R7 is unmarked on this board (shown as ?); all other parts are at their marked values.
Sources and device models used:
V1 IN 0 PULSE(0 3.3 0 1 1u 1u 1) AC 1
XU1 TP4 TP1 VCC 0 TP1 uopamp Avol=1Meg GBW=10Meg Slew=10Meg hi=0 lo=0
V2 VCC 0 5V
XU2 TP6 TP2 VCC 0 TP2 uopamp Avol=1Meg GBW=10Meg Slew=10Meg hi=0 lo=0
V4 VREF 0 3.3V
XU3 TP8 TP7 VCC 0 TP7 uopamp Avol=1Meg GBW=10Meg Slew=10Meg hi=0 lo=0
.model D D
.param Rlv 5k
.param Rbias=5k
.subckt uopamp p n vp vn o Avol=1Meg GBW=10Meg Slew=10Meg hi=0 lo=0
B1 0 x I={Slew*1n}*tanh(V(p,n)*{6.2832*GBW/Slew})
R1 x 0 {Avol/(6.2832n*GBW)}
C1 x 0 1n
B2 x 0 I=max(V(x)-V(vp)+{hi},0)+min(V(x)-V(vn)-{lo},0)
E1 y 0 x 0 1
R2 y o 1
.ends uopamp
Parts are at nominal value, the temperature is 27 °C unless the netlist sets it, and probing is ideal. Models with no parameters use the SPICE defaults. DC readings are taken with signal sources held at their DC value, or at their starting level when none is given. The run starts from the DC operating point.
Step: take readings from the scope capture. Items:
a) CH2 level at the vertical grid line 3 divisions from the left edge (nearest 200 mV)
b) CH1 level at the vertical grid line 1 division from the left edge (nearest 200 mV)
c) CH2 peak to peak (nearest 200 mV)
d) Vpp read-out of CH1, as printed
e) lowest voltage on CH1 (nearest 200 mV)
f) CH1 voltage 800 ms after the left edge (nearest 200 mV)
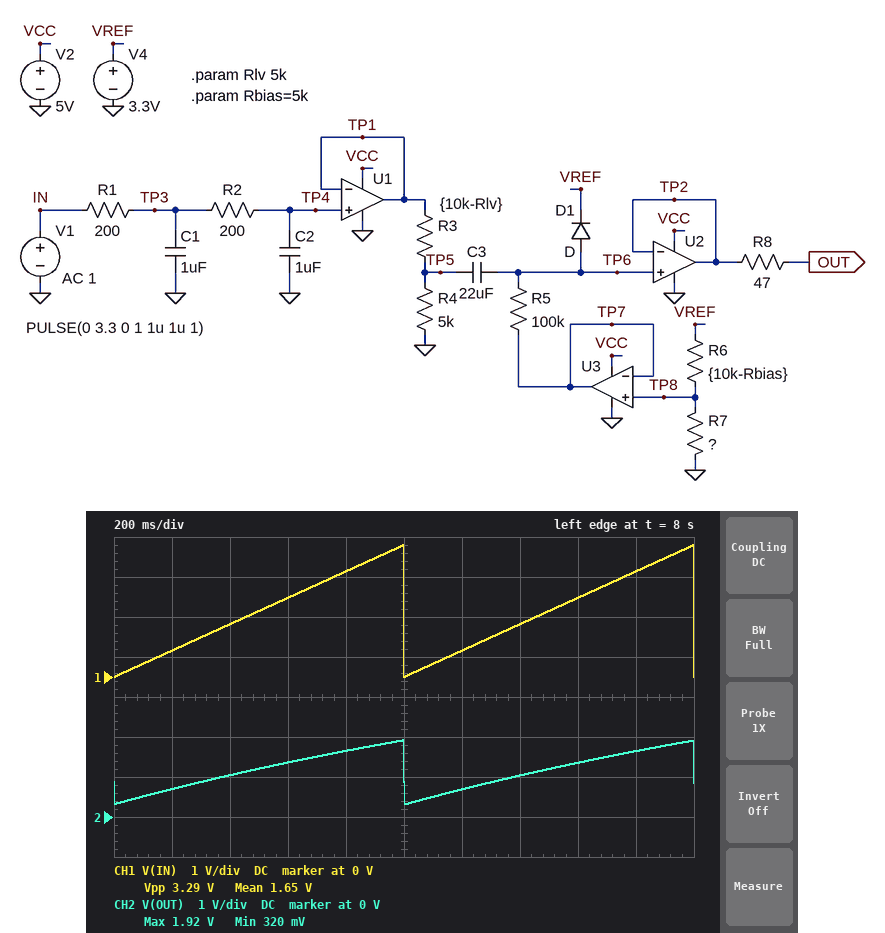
1.4 V
600 mV
1.6 V
3.29 V
0 V
2.6 V
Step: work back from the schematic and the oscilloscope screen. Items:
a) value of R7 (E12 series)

2.7 kΩ
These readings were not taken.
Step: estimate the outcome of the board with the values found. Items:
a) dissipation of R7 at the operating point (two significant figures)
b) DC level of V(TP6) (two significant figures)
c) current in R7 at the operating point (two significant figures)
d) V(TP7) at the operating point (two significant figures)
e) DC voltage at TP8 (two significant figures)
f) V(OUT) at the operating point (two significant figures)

500 µW
1.2 V
430 µA
1.2 V
1.2 V
1.2 V
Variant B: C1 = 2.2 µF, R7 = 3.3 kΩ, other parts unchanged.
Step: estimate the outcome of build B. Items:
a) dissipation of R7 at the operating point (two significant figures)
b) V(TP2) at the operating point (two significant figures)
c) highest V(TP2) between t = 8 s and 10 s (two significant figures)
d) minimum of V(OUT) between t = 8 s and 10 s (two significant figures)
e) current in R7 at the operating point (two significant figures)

520 µW
1.3 V
2.1 V
470 mV
400 µA
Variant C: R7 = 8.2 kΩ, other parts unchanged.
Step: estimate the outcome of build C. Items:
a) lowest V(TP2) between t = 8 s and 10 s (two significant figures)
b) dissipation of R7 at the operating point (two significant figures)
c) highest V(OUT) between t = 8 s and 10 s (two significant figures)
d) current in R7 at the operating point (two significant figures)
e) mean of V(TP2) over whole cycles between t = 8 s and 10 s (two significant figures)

1.2 V
510 µW
2.8 V
250 µA
2.1 V
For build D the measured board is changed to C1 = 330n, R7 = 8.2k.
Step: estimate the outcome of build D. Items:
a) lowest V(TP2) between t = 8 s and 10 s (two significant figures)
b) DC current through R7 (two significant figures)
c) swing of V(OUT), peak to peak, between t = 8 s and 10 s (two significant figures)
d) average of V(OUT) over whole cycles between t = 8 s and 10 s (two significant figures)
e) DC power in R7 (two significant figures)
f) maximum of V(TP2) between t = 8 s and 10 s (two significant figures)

1.2 V
250 µA
1.6 V
2.1 V
510 µW
2.8 V
